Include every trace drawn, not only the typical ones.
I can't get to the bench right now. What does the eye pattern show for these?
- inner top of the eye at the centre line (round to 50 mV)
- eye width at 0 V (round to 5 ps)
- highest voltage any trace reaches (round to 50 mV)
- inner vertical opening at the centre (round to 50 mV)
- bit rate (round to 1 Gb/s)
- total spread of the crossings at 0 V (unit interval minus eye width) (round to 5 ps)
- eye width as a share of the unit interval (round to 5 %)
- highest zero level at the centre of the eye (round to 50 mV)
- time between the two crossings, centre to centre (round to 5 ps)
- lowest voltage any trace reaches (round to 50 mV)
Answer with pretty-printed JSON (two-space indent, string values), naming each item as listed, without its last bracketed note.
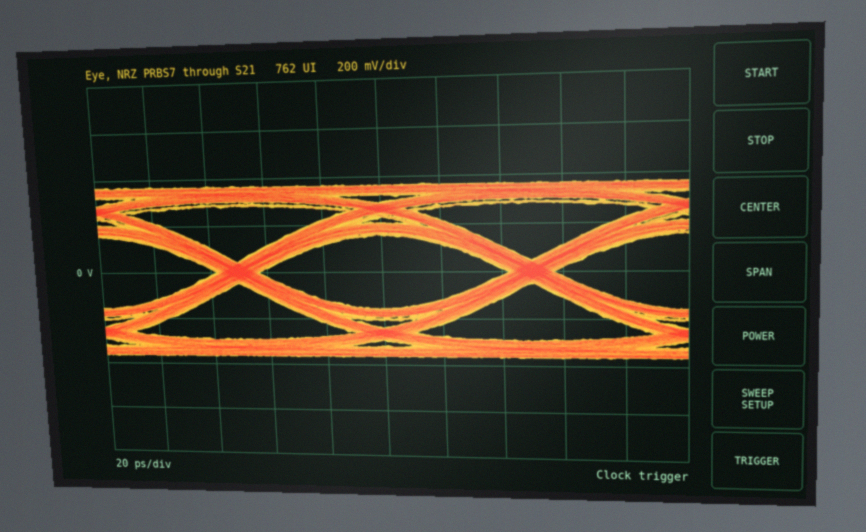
{
  "inner top of the eye at the centre line": "150 mV",
  "eye width at 0 V": "85 ps",
  "highest voltage any trace reaches": "350 mV",
  "inner vertical opening at the centre": "300 mV",
  "bit rate": "10 Gb/s",
  "total spread of the crossings at 0 V (unit interval minus eye width)": "15 ps",
  "eye width as a share of the unit interval": "85 %",
  "highest zero level at the centre of the eye": "-150 mV",
  "time between the two crossings, centre to centre": "100 ps",
  "lowest voltage any trace reaches": "-350 mV"
}
